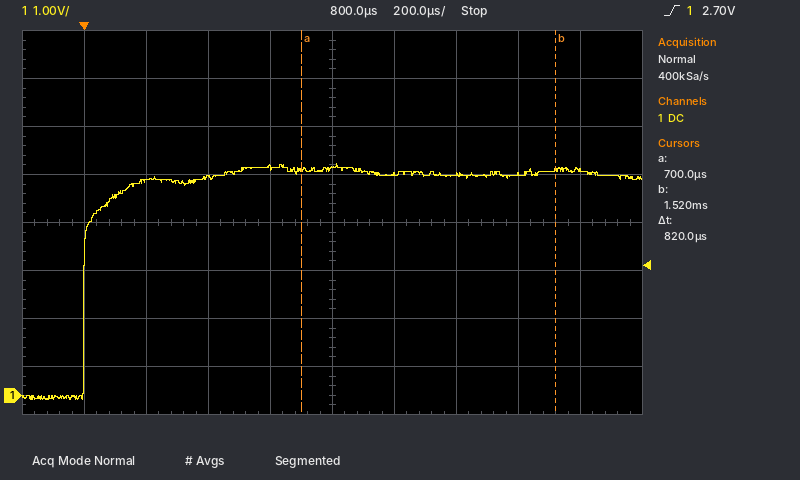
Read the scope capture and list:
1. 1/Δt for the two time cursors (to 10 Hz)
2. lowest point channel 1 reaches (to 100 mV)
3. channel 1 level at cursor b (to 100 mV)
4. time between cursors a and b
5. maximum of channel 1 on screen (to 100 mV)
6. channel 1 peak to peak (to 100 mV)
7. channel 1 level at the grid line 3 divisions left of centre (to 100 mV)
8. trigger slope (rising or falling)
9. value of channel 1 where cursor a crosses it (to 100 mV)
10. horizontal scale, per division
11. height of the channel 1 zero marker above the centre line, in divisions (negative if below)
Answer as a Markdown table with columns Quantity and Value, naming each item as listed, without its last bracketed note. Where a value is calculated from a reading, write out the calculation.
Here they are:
| Quantity | Value |
|---|---|
| 1/Δt for the two time cursors | 1 / 820 µs ≈ 1.22 kHz |
| lowest point channel 1 reaches | -100 mV |
| channel 1 level at cursor b | 4.7 V |
| time between cursors a and b | 820 µs |
| maximum of channel 1 on screen | 4.8 V |
| channel 1 peak to peak | 4.8 V − (-100 mV) = 4.9 V |
| channel 1 level at the grid line 3 divisions left of centre | 4.5 V |
| trigger slope | rising |
| value of channel 1 where cursor a crosses it | 4.7 V |
| horizontal scale, per division | 200 µs |
| height of the channel 1 zero marker above the centre line, in divisions | -3.6 div |
